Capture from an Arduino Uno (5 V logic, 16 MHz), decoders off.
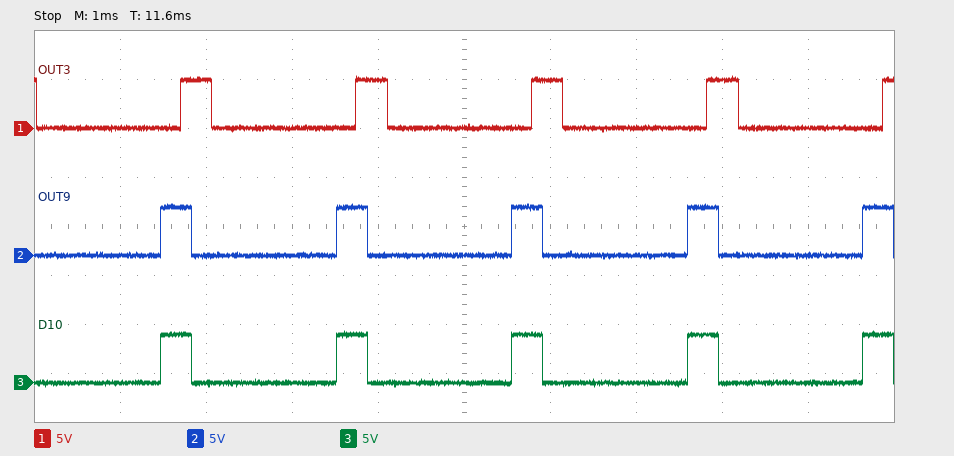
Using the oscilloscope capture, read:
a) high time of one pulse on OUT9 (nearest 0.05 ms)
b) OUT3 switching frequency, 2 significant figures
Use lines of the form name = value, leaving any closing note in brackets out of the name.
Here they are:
high time of one pulse on OUT9 = 0.35 ms
OUT3 switching frequency, 2 significant figures = 490 Hz
